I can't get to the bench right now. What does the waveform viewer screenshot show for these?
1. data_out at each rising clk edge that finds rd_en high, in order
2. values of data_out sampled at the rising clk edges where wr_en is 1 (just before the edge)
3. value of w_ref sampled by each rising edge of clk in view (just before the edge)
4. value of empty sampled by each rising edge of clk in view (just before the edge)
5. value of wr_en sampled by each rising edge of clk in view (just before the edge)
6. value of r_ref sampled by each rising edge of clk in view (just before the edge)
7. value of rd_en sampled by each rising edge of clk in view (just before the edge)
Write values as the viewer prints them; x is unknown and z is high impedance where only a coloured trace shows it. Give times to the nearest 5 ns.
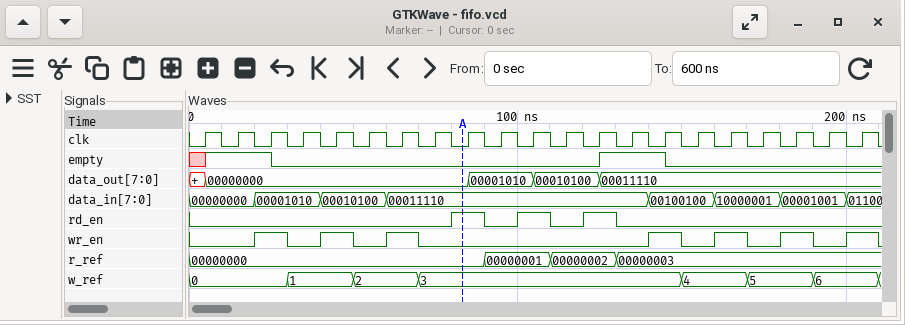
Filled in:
00000000, 00001010, 00010100
00000000, 00000000, 00000000, 00011110, 00011110, 00011110, 00011110
0, 0, 0, 1, 1, 2, 2, 3, 3, 3, 3, 3, 3, 3, 3, 4, 4, 5, 5, 6, 6
x 1 1 0 0 0 0 0 0 0 0 0 0 1 1 0 0 0 0 0 0
0 0 1 0 1 0 1 0 0 0 0 0 0 0 1 0 1 0 1 0 1
00000000, 00000000, 00000000, 00000000, 00000000, 00000000, 00000000, 00000000, 00000000, 00000001, 00000001, 00000002, 00000002, 00000003, 00000003, 00000003, 00000003, 00000003, 00000003, 00000003, 00000003
0 0 0 0 0 0 0 0 1 0 1 0 1 0 0 0 0 0 0 0 0
